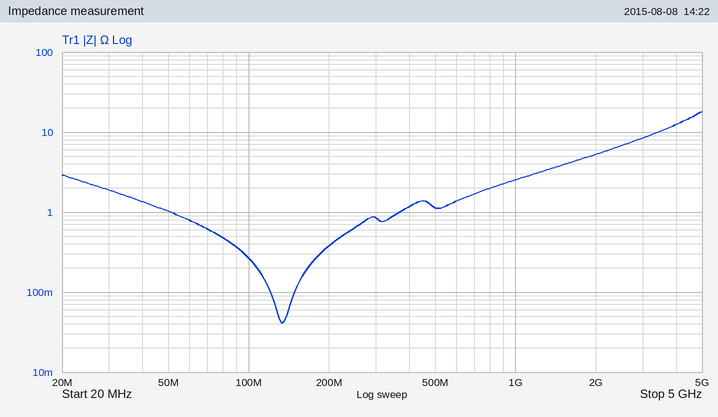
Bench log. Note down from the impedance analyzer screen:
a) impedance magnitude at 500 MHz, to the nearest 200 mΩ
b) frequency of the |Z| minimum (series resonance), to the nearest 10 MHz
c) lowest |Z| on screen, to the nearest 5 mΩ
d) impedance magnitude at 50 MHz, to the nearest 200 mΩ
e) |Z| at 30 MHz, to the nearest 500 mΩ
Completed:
1.2 Ω
130 MHz
40 mΩ
1.0 Ω
2.0 Ω
